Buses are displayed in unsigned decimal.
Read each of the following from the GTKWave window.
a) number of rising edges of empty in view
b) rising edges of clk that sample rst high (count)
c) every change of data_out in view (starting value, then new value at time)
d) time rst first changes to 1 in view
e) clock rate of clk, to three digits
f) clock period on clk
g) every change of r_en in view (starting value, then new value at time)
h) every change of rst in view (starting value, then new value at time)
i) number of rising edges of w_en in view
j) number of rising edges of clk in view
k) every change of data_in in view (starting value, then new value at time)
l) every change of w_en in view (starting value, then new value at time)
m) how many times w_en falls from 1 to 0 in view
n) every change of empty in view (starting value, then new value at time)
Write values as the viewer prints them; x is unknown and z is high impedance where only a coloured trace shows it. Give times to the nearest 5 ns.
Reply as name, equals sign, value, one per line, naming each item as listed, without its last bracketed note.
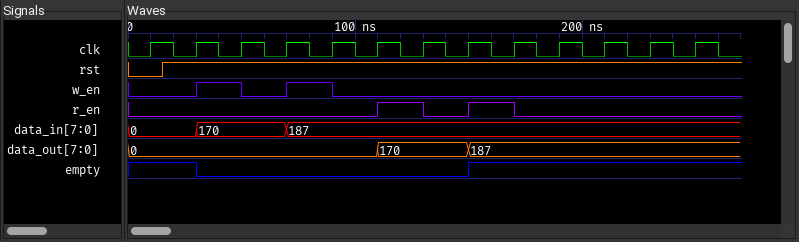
number of rising edges of empty in view = 1
rising edges of clk that sample rst high = 12
every change of data_out in view = 0, 170 at 110 ns, 187 at 150 ns
time rst first changes to 1 in view = 15 ns
clock rate of clk, to three digits = 50.0 MHz
clock period on clk = 20 ns
every change of r_en in view = 0, 1 at 110 ns, 0 at 130 ns, 1 at 150 ns, 0 at 170 ns
every change of rst in view = 0, 1 at 15 ns
number of rising edges of w_en in view = 2
number of rising edges of clk in view = 13
every change of data_in in view = 0, 170 at 30 ns, 187 at 70 ns
every change of w_en in view = 0, 1 at 30 ns, 0 at 50 ns, 1 at 70 ns, 0 at 90 ns
how many times w_en falls from 1 to 0 in view = 2
every change of empty in view = 1, 0 at 30 ns, 1 at 150 ns
